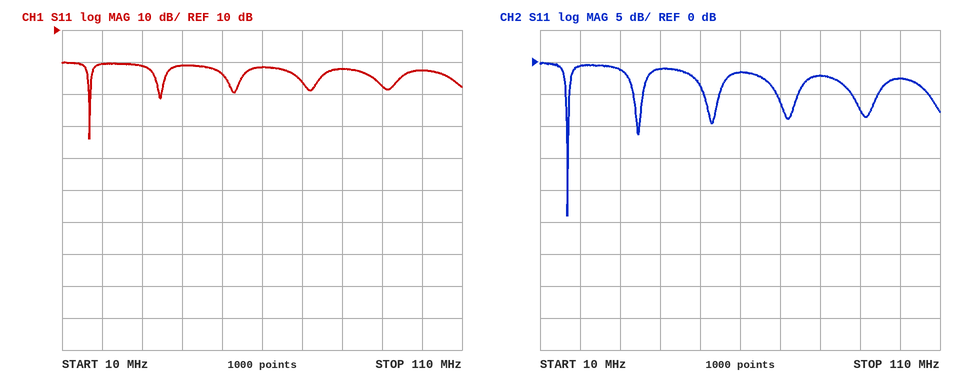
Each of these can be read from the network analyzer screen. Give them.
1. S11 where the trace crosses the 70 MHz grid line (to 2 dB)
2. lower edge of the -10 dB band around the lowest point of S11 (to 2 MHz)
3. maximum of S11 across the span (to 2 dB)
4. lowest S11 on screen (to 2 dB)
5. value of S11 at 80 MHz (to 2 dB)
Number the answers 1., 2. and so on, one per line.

1. -6 dB
2. 16 MHz
3. 0 dB
4. -24 dB
5. -2 dB
